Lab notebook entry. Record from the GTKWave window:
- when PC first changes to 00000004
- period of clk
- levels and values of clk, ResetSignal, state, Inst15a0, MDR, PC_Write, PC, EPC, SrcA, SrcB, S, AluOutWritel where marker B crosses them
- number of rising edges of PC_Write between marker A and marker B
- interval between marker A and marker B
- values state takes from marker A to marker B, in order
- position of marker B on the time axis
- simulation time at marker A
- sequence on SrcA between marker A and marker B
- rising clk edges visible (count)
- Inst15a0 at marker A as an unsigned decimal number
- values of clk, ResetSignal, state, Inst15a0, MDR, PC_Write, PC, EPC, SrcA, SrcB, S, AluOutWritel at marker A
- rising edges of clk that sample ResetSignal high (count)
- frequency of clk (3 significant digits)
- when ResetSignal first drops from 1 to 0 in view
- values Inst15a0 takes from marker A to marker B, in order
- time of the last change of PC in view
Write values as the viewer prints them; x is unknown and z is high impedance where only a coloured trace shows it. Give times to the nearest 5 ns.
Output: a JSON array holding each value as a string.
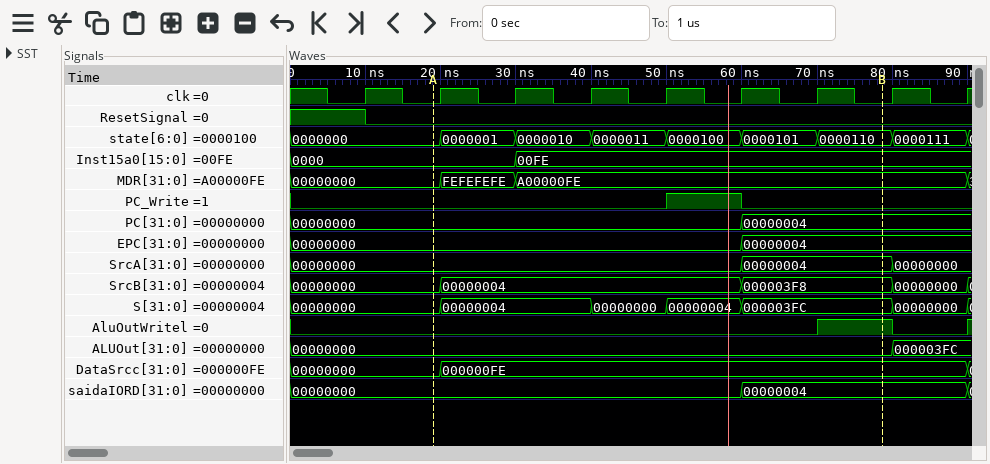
["60 ns", "10 ns", "clk=0, ResetSignal=0, state=0000110, Inst15a0=00FE, MDR=A00000FE, PC_Write=0, PC=00000004, EPC=00000004, SrcA=00000004, SrcB=000003F8, S=000003FC, AluOutWritel=1", "1", "60 ns", "0000000, 0000001, 0000010, 0000011, 0000100, 0000101, 0000110", "80 ns", "20 ns", "00000000, 00000004", "9", "0", "clk=0, ResetSignal=0, state=0000000, Inst15a0=0000, MDR=00000000, PC_Write=0, PC=00000000, EPC=00000000, SrcA=00000000, SrcB=00000000, S=00000000, AluOutWritel=0", "1", "100 MHz", "10 ns", "0000, 00FE", "60 ns"]
